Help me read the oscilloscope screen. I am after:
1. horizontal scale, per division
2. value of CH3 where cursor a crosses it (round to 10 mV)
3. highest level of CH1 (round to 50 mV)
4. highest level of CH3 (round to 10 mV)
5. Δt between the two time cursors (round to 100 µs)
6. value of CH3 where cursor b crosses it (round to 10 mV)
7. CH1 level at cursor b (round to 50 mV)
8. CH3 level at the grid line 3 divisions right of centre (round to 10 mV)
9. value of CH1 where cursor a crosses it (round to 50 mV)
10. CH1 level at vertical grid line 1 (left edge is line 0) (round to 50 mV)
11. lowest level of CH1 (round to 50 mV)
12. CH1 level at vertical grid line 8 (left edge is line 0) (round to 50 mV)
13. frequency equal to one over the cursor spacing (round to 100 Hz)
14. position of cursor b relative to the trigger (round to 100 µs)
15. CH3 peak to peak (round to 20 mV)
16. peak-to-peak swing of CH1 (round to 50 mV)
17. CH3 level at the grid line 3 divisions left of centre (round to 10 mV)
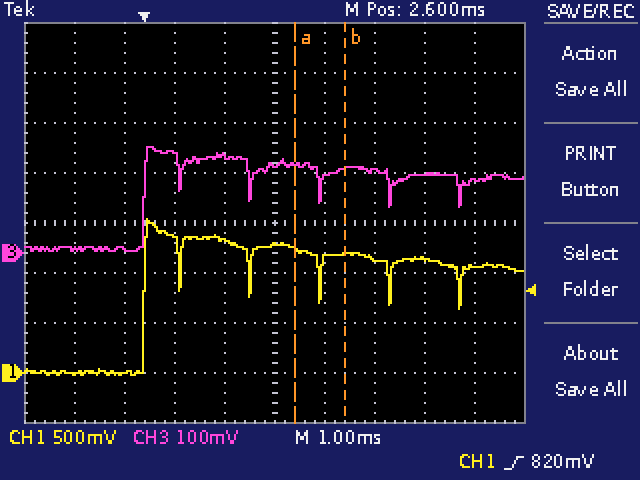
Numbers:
1 ms
180 mV
1.55 V
210 mV
1.0 ms
170 mV
1.20 V
160 mV
1.25 V
0 mV
0 mV
1.15 V
1.0 kHz
+4.0 ms
200 mV
1.55 V
10 mV
